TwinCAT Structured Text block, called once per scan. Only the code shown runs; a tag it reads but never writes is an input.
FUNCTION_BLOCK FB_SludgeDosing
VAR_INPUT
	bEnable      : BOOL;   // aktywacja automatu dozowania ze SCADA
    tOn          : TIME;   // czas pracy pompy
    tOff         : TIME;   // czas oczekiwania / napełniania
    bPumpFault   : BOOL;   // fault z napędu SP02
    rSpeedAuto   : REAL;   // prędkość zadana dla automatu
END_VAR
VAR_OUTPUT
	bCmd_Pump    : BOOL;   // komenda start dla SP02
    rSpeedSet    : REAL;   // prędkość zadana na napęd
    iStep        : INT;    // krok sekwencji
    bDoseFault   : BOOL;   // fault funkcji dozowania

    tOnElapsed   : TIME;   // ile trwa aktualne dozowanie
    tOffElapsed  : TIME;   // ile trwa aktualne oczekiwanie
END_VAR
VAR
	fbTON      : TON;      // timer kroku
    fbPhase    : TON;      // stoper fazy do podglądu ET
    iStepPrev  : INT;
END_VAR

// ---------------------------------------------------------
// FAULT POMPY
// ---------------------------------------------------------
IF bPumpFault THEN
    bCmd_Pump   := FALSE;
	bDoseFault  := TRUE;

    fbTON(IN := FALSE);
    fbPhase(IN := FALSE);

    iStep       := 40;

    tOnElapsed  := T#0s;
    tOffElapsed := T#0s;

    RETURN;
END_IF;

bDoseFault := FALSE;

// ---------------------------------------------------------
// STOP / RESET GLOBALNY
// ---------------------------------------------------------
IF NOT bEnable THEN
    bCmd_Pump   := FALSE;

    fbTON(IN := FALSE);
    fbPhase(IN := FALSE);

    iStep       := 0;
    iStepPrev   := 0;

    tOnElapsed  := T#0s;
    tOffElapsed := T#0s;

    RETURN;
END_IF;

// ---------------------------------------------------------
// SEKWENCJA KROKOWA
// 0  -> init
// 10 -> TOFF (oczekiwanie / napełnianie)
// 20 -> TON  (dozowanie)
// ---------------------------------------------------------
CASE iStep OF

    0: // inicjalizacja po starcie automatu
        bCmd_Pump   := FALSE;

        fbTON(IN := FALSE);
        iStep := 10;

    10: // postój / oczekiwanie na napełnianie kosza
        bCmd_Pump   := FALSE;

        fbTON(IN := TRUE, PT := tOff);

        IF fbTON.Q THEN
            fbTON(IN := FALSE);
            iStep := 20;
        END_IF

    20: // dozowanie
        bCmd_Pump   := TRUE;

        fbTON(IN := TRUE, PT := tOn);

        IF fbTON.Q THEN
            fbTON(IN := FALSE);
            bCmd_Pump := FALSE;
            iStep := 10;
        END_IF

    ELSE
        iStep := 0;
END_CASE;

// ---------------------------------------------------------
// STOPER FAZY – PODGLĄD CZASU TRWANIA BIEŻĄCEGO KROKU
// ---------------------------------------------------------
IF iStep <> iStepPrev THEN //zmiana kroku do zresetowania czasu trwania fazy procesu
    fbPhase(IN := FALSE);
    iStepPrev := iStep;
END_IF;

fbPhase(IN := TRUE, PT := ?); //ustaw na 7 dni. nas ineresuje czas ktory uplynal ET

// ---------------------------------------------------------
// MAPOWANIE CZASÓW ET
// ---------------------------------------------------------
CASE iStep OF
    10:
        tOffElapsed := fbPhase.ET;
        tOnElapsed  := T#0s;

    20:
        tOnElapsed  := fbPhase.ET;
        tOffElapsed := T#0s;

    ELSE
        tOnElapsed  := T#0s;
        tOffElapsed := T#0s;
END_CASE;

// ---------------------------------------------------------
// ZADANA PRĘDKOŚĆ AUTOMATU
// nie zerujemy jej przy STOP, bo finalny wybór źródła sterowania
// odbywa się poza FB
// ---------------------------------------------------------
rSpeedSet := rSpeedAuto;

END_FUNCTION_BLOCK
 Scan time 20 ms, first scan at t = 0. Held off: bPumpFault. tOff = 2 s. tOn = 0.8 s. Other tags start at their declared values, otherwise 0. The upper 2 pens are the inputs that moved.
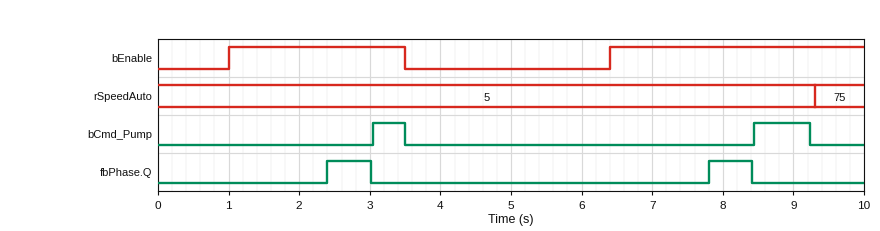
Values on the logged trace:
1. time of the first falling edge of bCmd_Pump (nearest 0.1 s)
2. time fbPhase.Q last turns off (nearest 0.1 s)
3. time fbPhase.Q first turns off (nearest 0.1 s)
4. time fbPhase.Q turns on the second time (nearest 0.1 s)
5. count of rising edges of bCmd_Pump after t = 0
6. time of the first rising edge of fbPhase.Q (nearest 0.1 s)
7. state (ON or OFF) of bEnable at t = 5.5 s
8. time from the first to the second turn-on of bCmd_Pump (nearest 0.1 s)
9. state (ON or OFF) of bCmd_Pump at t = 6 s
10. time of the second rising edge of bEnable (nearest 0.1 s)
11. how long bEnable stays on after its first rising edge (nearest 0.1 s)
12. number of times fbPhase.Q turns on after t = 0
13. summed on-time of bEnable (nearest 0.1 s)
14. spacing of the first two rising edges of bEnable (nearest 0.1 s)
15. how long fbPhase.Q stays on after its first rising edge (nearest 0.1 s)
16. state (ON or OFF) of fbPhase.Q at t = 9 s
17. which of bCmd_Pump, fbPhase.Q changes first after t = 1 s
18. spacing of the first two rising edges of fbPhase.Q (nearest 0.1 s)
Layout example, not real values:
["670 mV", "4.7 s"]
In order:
["3.5 s", "8.4 s", "3.0 s", "7.8 s", "2", "2.4 s", "OFF", "5.4 s", "OFF", "6.4 s", "2.5 s", "2", "6.1 s", "5.4 s", "0.6 s", "OFF", "fbPhase.Q", "5.4 s"]
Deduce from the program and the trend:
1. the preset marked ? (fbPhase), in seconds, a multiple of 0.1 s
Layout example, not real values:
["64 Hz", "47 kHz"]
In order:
["1.4 s"]
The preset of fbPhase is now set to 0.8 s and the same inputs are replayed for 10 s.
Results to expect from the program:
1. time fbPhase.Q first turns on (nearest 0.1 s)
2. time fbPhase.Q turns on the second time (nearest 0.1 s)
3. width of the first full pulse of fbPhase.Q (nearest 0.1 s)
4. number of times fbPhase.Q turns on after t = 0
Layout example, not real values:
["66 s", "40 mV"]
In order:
["1.8 s", "7.2 s", "1.2 s", "3"]
